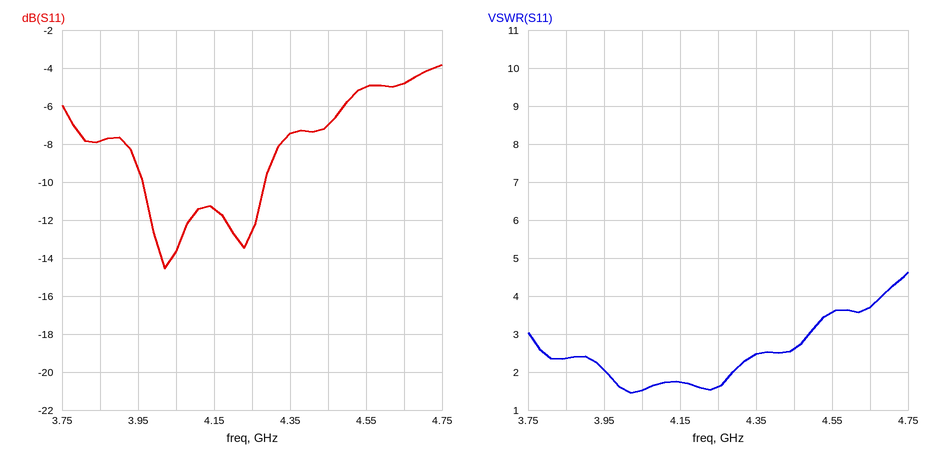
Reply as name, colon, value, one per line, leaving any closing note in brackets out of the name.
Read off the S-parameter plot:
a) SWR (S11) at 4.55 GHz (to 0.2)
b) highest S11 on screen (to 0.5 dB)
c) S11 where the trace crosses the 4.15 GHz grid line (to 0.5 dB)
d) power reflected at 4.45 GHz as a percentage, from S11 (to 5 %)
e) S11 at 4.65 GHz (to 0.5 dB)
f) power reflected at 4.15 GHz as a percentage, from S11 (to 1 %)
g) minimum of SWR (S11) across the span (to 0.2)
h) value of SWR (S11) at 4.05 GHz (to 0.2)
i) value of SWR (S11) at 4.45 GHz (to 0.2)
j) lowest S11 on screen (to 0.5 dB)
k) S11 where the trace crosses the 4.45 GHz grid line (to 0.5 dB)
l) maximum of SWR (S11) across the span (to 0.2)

SWR (S11) at 4.55 GHz: 3.6
highest S11 on screen: -4.0 dB
S11 where the trace crosses the 4.15 GHz grid line: -11.5 dB
power reflected at 4.45 GHz as a percentage, from S11: 20 %
S11 at 4.65 GHz: -5.0 dB
power reflected at 4.15 GHz as a percentage, from S11: 7 %
minimum of SWR (S11) across the span: 1.4
value of SWR (S11) at 4.05 GHz: 1.6
value of SWR (S11) at 4.45 GHz: 2.6
lowest S11 on screen: -14.5 dB
S11 where the trace crosses the 4.45 GHz grid line: -7.0 dB
maximum of SWR (S11) across the span: 4.6
